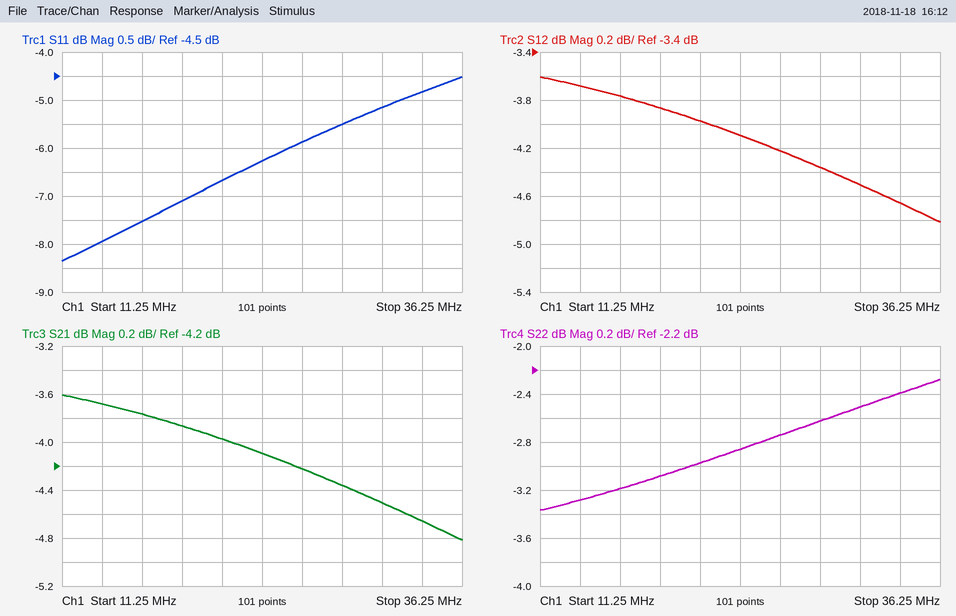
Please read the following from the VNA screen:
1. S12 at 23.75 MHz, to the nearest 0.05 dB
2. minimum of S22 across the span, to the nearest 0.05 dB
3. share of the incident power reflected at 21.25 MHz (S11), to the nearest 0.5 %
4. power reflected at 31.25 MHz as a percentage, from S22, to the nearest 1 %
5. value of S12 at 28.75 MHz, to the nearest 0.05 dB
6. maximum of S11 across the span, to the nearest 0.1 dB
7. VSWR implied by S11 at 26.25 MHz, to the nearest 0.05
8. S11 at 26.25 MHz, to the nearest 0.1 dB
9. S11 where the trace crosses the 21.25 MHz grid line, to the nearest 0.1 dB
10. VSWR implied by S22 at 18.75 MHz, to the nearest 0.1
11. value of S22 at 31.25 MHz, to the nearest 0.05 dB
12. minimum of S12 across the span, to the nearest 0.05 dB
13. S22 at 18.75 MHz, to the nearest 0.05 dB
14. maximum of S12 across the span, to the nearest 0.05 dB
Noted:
-4.10 dB
-3.35 dB
21.5 %
56 %
-4.35 dB
-4.5 dB
3.05
-5.9 dB
-6.7 dB
5.7
-2.50 dB
-4.80 dB
-3.10 dB
-3.60 dB
